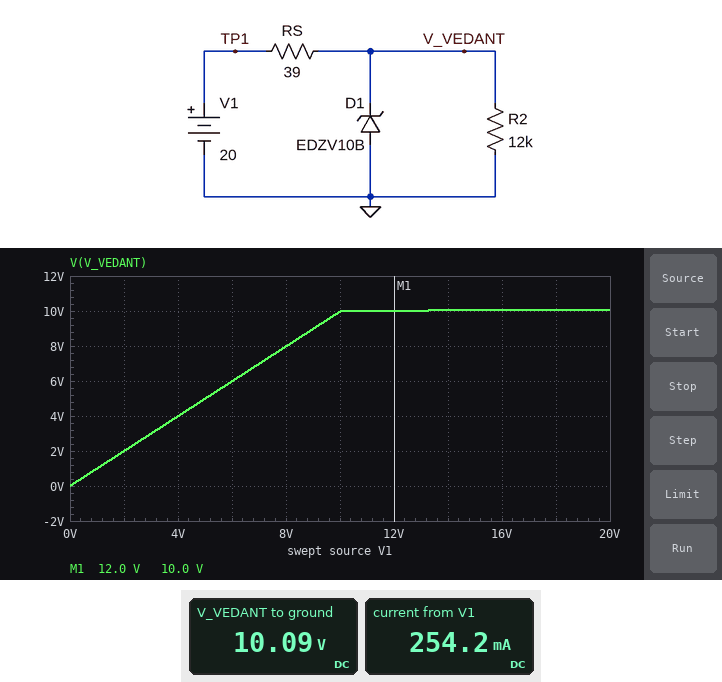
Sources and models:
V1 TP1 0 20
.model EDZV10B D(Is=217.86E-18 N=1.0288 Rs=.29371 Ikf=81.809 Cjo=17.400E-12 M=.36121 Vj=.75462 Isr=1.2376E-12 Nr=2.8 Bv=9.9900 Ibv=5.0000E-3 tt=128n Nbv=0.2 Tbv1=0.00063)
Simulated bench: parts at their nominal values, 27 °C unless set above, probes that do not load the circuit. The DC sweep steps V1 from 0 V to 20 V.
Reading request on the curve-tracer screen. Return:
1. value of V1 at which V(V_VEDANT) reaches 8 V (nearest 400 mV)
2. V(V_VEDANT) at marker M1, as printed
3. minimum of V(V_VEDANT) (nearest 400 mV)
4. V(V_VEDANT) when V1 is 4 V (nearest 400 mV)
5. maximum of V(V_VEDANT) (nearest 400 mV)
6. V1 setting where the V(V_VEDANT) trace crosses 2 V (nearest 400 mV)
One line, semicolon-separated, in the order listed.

8.0 V; 10.0 V; 0 V; 4.0 V; 10.0 V; 2.0 V
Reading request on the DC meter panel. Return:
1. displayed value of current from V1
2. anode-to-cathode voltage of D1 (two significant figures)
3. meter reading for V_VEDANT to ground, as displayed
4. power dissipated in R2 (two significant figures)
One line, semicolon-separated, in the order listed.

254.2 mA; -10 V; 10.09 V; 8.5 mW
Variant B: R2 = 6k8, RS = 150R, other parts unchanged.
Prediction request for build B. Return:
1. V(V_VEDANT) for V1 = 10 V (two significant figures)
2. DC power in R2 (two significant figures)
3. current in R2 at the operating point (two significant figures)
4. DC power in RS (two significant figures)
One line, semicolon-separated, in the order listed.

9.8 V; 15 mW; 1.5 mA; 660 mW
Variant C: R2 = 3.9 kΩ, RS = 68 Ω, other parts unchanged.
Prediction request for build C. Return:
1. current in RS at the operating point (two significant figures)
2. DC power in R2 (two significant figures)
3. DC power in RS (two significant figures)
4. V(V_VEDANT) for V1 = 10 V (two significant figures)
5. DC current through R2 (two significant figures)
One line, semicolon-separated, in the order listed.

150 mA; 26 mW; 1.5 W; 9.8 V; 2.6 mA
